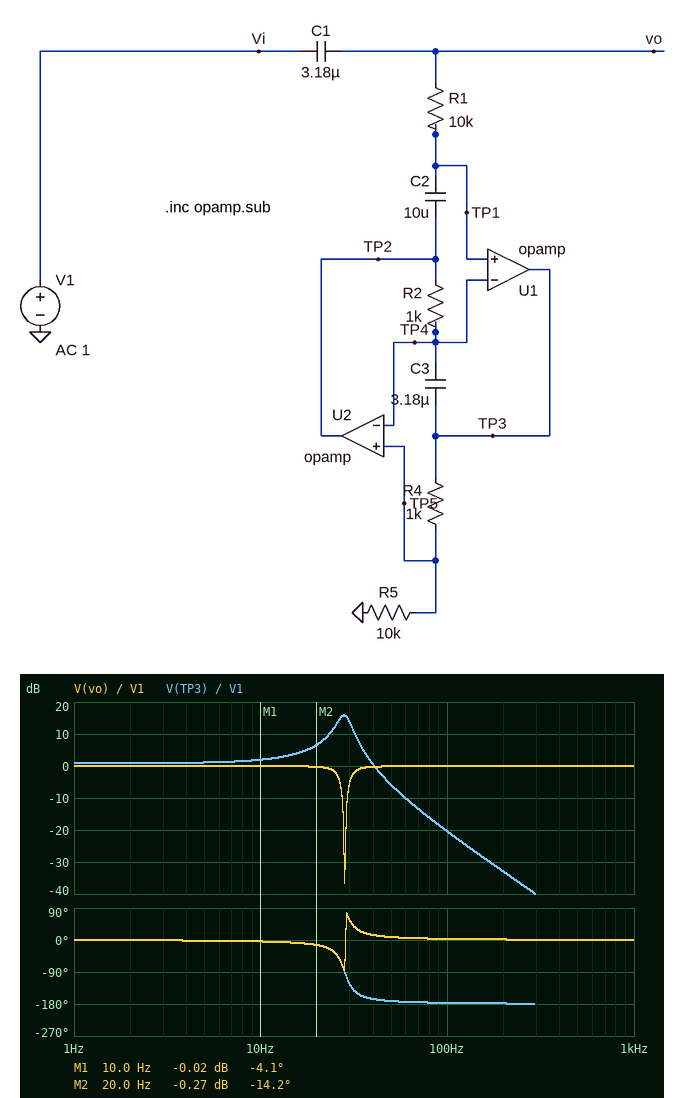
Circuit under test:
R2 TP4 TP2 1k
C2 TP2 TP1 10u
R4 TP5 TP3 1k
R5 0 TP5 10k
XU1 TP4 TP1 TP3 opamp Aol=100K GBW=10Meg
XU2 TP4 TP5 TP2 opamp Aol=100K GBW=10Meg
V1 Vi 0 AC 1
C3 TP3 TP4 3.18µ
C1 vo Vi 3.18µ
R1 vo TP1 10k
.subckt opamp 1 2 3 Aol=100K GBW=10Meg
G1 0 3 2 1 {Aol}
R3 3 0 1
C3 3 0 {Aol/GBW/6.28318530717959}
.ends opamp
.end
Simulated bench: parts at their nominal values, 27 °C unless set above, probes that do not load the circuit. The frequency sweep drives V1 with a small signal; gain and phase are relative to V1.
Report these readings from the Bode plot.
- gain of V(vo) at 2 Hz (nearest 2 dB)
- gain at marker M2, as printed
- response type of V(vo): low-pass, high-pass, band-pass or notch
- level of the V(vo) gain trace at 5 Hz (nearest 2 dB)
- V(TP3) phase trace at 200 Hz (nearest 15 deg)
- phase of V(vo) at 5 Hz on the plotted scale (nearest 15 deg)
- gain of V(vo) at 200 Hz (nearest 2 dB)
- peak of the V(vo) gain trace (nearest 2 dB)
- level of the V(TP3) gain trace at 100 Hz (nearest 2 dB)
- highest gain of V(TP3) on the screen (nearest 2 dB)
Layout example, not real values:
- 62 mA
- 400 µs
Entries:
- 0 dB
- -0.27 dB
- notch
- 0 dB
- -180 deg
- 0 deg
- 0 dB
- 0 dB
- -20 dB
- 16 dB
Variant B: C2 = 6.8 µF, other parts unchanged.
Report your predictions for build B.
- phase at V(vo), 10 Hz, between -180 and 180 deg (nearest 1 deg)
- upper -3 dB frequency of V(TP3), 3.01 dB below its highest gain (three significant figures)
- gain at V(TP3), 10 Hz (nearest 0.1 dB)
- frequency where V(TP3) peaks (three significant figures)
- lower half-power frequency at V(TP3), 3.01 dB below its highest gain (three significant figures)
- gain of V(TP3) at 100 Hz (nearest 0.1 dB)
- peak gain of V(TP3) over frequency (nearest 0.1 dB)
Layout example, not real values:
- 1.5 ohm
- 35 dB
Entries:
- -3 deg
- 36.5 Hz
- 1.6 dB
- 34.0 Hz
- 31.4 Hz
- -16.7 dB
- 17.5 dB
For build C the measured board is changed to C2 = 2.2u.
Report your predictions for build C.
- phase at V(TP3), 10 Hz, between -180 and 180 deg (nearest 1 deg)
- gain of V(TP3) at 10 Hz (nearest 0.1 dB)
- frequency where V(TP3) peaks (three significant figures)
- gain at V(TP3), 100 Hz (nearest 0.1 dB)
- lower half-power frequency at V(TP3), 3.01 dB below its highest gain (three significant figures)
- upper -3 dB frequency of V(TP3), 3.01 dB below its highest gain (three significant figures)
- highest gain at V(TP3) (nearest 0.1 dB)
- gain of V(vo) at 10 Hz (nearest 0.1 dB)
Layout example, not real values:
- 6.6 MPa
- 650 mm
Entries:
- -1 deg
- 1.1 dB
- 60.1 Hz
- -4.1 dB
- 57.5 Hz
- 62.5 Hz
- 22.4 dB
- 0 dB
